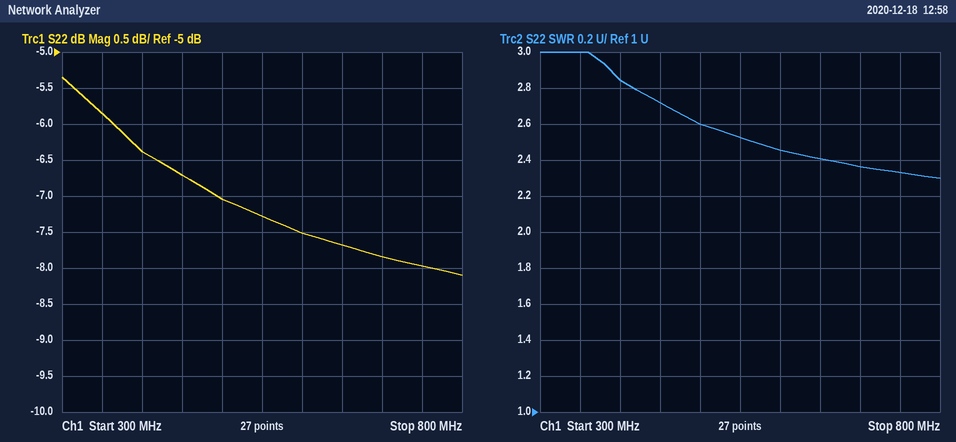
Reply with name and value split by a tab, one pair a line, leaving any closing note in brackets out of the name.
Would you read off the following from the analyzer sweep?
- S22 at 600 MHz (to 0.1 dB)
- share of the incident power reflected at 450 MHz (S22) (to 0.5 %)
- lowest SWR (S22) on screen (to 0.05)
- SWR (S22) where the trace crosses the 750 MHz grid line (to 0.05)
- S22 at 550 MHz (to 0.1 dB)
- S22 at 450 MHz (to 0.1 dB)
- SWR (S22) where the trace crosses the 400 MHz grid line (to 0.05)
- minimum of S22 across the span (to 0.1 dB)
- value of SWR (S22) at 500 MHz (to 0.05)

S22 at 600 MHz	-7.5 dB
share of the incident power reflected at 450 MHz (S22)	21.5 %
lowest SWR (S22) on screen	2.30
SWR (S22) where the trace crosses the 750 MHz grid line	2.35
S22 at 550 MHz	-7.3 dB
S22 at 450 MHz	-6.7 dB
SWR (S22) where the trace crosses the 400 MHz grid line	2.85
minimum of S22 across the span	-8.1 dB
value of SWR (S22) at 500 MHz	2.60
